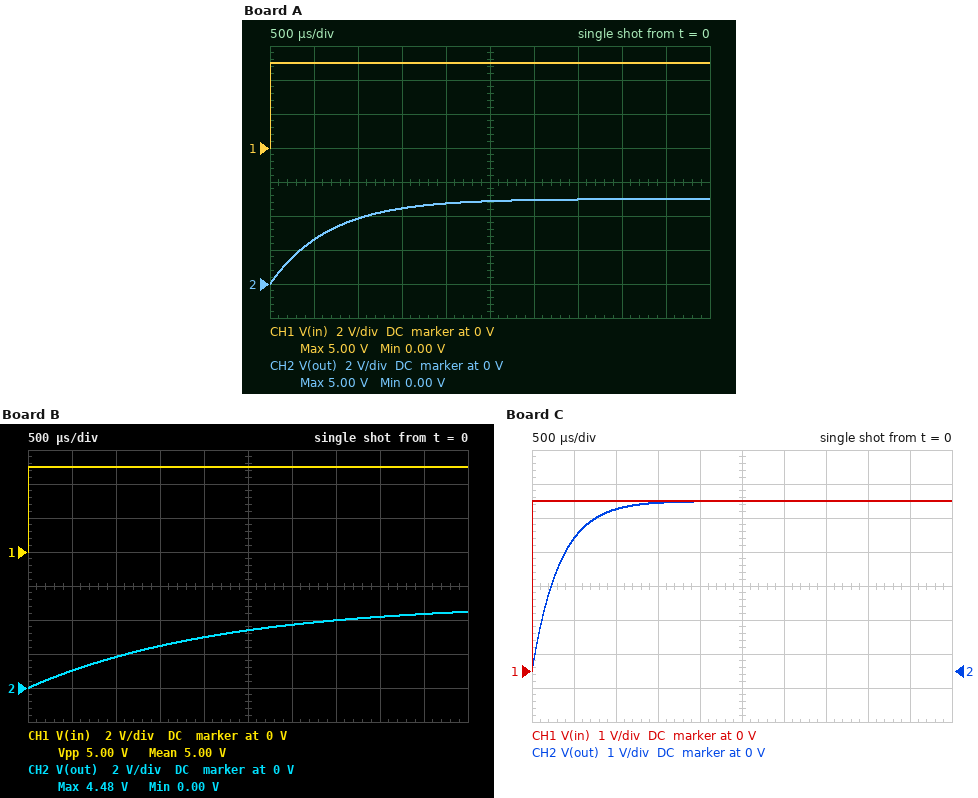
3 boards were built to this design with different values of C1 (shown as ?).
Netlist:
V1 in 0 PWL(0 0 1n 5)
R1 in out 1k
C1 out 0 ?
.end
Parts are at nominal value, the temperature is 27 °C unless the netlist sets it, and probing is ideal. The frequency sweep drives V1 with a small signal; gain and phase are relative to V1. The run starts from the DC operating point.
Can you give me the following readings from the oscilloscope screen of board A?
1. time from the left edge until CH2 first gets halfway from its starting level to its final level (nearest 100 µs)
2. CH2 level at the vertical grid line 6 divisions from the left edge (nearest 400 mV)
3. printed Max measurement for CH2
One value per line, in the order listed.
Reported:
500 µs
4.8 V
5.00 V
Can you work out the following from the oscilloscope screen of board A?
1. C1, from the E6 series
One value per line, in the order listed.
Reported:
680 nF
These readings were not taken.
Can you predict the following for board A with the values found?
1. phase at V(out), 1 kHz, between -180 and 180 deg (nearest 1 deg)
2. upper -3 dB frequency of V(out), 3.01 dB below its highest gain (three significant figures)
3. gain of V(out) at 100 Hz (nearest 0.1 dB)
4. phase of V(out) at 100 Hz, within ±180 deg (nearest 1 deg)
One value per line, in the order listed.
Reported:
-77 deg
234 Hz
-0.7 dB
-23 deg
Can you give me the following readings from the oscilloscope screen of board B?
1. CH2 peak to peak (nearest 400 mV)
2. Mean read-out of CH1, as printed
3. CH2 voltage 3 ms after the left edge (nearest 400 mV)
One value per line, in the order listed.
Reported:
4.4 V
5.00 V
3.6 V
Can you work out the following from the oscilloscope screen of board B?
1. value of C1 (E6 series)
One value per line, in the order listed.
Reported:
2.2 µF
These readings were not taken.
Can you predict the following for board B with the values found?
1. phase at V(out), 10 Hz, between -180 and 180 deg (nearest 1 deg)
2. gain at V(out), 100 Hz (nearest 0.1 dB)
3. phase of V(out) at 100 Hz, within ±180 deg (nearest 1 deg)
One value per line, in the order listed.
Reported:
-8 deg
-4.6 dB
-54 deg
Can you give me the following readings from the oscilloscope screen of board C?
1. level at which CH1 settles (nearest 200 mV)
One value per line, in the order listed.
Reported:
5.0 V
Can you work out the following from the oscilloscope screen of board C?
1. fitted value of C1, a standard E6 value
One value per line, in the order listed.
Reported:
330 nF
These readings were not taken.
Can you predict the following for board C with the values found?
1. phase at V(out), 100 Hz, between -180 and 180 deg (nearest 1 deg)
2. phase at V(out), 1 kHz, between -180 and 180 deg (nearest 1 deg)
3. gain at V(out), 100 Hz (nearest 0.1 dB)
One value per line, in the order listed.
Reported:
-12 deg
-64 deg
-0.2 dB
